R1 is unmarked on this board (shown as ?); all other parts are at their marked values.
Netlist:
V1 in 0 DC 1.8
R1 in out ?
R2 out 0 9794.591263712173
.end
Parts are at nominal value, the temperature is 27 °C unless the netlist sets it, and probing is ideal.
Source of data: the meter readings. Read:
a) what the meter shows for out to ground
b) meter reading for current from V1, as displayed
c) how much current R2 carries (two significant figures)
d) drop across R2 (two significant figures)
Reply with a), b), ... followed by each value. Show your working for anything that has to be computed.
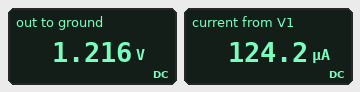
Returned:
a) 1.216 V
b) 124.2 µA
c) (1.216 V) / 9.795 kΩ = 120 µA
d) 1.216 V = 1.2 V
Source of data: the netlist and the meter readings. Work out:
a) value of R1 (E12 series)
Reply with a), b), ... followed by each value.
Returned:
a) 4.7 kΩ
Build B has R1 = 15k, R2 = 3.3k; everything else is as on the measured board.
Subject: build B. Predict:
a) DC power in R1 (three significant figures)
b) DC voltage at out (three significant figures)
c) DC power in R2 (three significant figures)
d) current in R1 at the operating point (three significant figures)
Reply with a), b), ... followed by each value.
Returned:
a) 145 µW
b) 325 mV
c) 31.9 µW
d) 98.4 µA
